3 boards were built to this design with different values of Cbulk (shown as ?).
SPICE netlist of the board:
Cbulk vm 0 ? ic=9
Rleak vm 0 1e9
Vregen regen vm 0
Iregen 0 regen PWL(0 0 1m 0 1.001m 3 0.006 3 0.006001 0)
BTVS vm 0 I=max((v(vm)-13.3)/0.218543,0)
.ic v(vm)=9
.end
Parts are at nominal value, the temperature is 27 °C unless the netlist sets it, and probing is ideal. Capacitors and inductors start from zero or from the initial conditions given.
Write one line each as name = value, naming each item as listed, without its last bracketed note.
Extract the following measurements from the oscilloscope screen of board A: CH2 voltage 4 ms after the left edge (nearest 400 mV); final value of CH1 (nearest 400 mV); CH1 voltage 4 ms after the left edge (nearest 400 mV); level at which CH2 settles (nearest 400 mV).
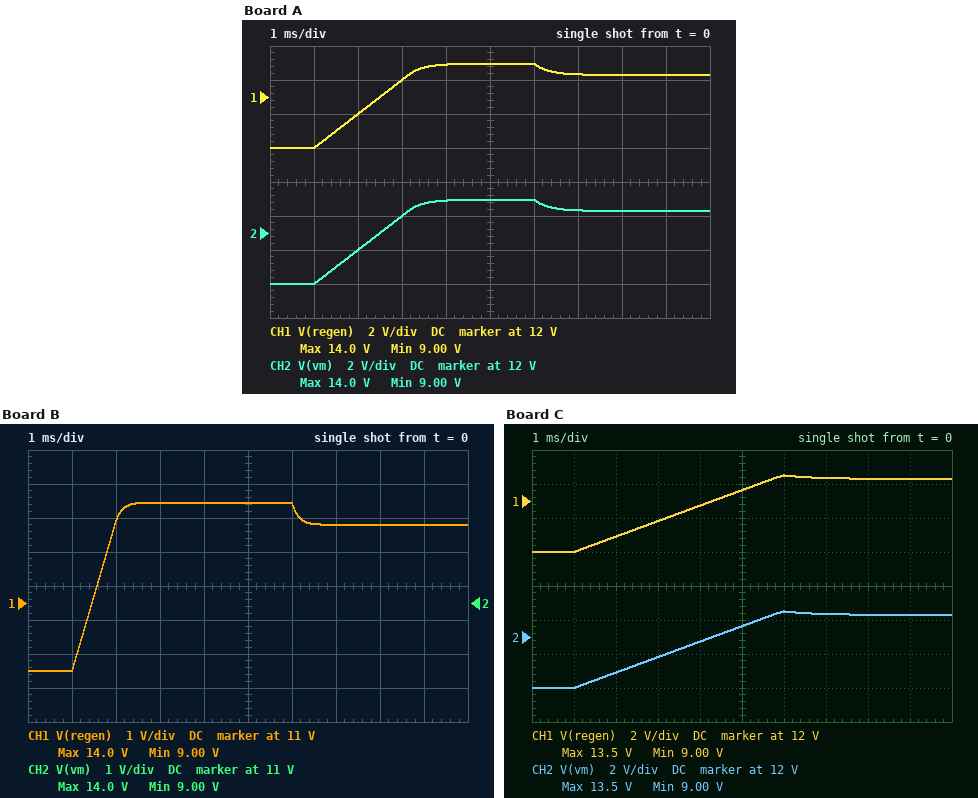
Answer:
CH2 voltage 4 ms after the left edge = 14.0 V
final value of CH1 = 13.2 V
CH1 voltage 4 ms after the left edge = 14.0 V
level at which CH2 settles = 13.2 V
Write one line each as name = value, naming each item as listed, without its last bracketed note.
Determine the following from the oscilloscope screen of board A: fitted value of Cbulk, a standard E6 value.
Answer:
fitted value of Cbulk, a standard E6 value = 1.5 mF
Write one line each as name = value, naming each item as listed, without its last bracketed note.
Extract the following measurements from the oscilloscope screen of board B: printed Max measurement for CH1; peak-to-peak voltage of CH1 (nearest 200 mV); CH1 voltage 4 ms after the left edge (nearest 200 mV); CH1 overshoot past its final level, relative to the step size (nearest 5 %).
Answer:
printed Max measurement for CH1 = 14.0 V
peak-to-peak voltage of CH1 = 5.0 V
CH1 voltage 4 ms after the left edge = 14.0 V
CH1 overshoot past its final level, relative to the step size = 15 %
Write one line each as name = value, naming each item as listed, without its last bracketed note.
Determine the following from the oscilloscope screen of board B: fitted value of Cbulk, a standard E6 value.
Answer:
fitted value of Cbulk, a standard E6 value = 680 µF
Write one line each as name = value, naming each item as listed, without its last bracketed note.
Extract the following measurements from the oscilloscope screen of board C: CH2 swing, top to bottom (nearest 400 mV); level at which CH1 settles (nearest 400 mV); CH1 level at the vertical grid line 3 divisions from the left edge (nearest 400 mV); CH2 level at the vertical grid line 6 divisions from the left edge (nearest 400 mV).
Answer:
CH2 swing, top to bottom = 4.4 V
level at which CH1 settles = 13.2 V
CH1 level at the vertical grid line 3 divisions from the left edge = 10.8 V
CH2 level at the vertical grid line 6 divisions from the left edge = 13.6 V
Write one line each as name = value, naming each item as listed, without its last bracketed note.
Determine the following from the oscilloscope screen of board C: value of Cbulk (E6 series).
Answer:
value of Cbulk = 3.3 mF
